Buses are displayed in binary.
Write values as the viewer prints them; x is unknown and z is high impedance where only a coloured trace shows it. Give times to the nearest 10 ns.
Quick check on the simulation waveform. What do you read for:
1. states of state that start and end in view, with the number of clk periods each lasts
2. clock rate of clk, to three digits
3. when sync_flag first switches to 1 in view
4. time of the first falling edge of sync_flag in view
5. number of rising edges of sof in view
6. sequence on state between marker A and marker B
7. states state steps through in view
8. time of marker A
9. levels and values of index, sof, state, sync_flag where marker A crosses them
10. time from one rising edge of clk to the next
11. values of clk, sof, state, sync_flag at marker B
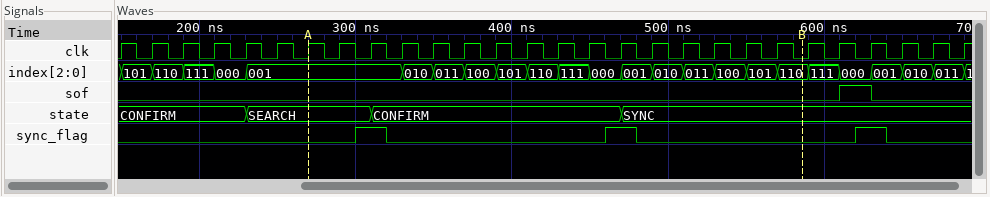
SEARCH: 4, CONFIRM: 8
50.0 MHz
300 ns
320 ns
1
SEARCH, CONFIRM, SYNC
CONFIRM, SEARCH, CONFIRM, SYNC
270 ns
index=001, sof=0, state=SEARCH, sync_flag=0
20 ns
clk=0, sof=0, state=SYNC, sync_flag=0
